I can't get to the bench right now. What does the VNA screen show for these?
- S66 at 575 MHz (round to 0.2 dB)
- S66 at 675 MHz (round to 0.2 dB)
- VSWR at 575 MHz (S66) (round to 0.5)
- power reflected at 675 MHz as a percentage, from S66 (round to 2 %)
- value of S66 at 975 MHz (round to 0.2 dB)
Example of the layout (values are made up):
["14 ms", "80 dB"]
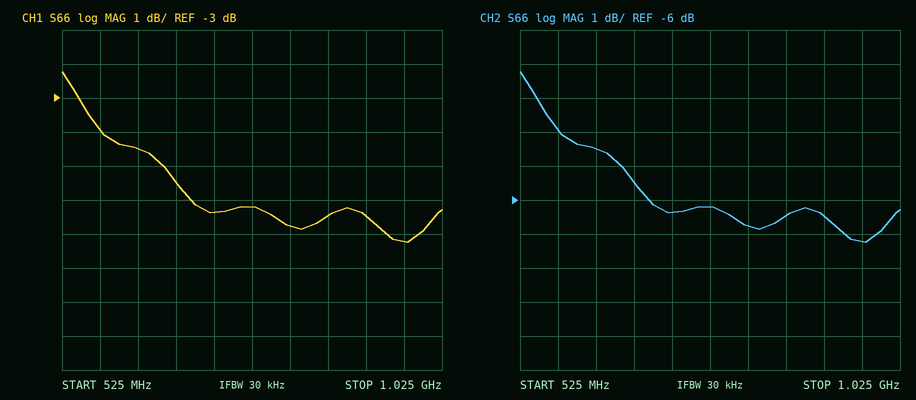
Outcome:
["-4.0 dB", "-5.4 dB", "4.5", "28 %", "-7.2 dB"]
